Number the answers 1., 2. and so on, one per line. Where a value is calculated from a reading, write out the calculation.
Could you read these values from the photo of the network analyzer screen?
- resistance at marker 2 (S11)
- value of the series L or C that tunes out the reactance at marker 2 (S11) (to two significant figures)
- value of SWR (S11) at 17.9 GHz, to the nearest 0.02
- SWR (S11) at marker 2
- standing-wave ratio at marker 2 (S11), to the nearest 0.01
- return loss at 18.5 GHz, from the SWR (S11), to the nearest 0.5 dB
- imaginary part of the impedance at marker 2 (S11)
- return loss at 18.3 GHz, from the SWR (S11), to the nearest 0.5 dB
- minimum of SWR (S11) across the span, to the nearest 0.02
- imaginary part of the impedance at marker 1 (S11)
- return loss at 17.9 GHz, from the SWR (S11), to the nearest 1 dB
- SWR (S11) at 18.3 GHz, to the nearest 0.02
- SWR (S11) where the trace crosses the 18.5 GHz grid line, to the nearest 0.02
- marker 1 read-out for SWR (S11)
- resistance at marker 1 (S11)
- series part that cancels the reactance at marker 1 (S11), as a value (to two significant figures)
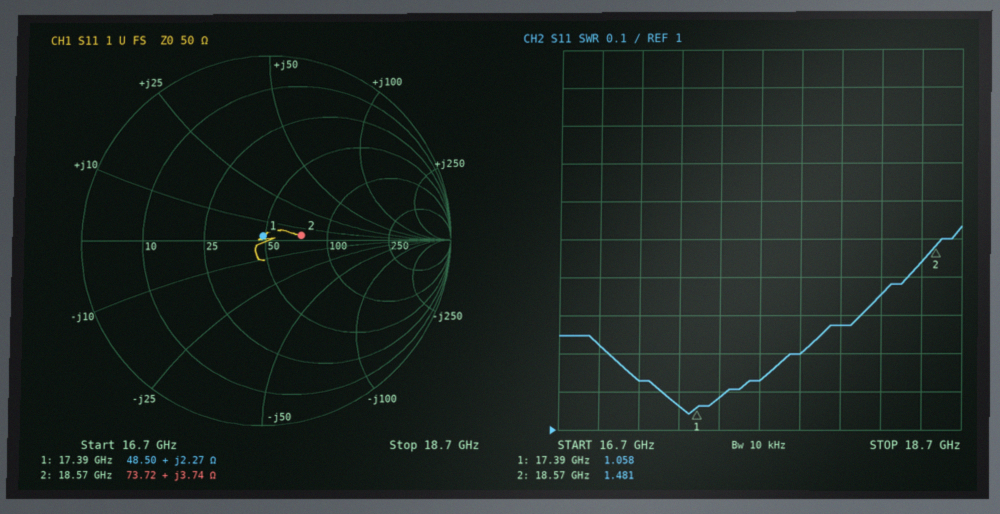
1. 73.72 Ω
2. C = 1/(2π × 18.57 GHz × 3.74 Ω) ≈ 2.3 pF
3. 1.20
4. 1.481
5. 1.48
6. −20 log10((1.44 − 1)/(1.44 + 1)) ≈ 14.9 dB, so 15.0 dB to the nearest 0.5 dB
7. +3.74 Ω
8. −20 log10((1.36 − 1)/(1.36 + 1)) ≈ 16.3 dB, so 16.5 dB to the nearest 0.5 dB
9. 1.04
10. +2.27 Ω
11. −20 log10((1.2 − 1)/(1.2 + 1)) ≈ 21 dB
12. 1.36
13. 1.44
14. 1.058
15. 48.50 Ω
16. C = 1/(2π × 17.39 GHz × 2.27 Ω) ≈ 4.0 pF
